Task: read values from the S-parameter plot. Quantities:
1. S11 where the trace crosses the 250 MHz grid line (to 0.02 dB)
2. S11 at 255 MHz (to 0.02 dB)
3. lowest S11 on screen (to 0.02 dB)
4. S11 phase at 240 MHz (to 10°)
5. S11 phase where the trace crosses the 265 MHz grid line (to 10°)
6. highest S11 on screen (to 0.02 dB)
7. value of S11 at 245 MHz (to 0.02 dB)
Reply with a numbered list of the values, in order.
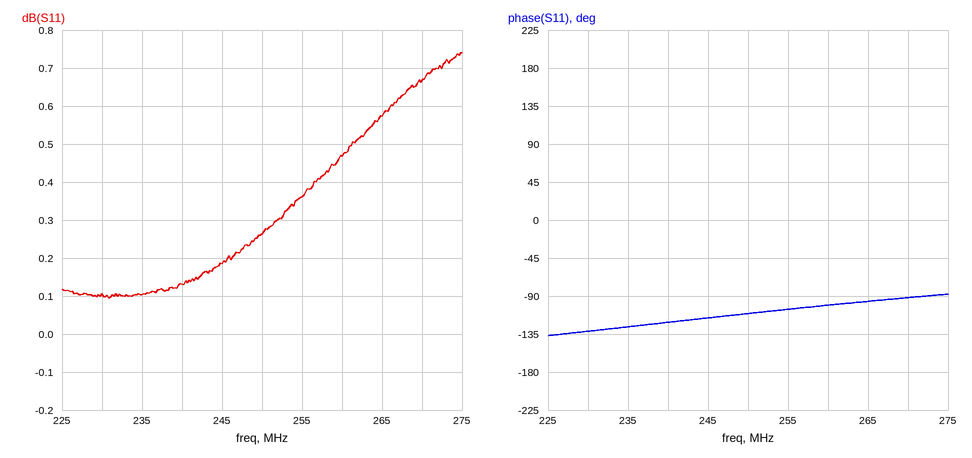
1. 0.26 dB
2. 0.36 dB
3. 0.10 dB
4. -120°
5. -100°
6. 0.74 dB
7. 0.18 dB
